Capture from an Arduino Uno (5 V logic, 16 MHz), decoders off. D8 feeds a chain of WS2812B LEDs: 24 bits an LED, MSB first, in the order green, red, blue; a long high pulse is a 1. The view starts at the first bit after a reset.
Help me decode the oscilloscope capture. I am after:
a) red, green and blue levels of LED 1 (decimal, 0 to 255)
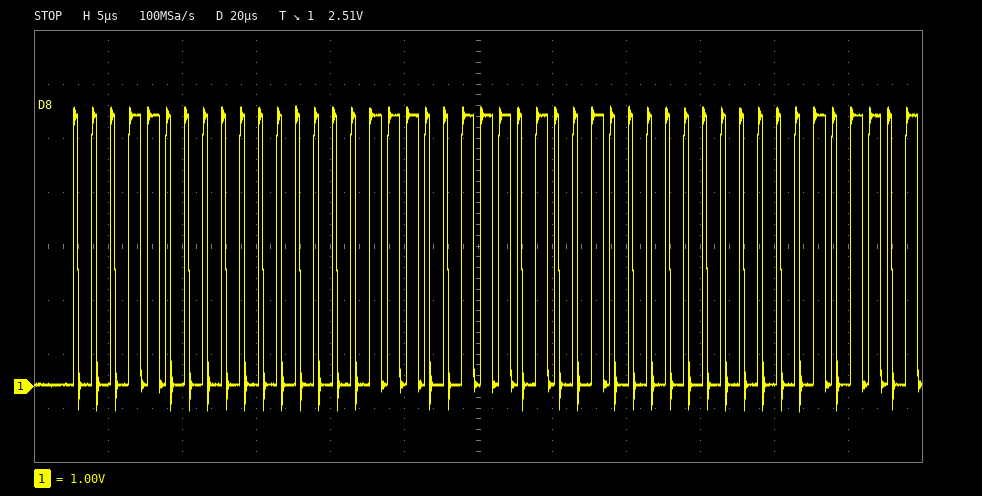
0, 24, 231
